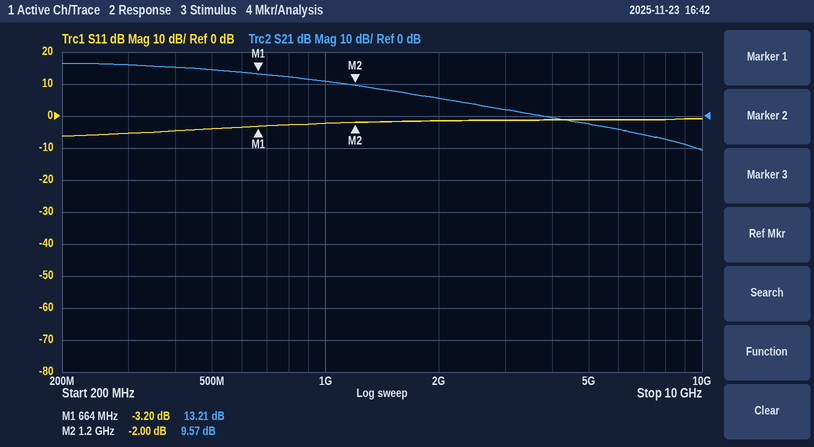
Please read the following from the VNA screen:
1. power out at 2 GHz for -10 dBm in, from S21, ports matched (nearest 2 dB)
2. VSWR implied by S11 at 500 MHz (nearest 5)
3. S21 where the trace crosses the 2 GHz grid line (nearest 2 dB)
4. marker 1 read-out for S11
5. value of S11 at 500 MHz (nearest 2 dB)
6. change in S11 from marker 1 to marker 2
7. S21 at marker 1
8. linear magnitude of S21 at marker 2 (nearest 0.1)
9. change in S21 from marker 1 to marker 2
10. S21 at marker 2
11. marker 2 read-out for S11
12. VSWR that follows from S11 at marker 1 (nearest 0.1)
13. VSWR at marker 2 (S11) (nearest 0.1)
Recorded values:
-4 dBm
5
6 dB
-3.20 dB
-4 dB
1.20 dB
13.21 dB
3.0
-3.64 dB
9.57 dB
-2.00 dB
5.5
8.7
